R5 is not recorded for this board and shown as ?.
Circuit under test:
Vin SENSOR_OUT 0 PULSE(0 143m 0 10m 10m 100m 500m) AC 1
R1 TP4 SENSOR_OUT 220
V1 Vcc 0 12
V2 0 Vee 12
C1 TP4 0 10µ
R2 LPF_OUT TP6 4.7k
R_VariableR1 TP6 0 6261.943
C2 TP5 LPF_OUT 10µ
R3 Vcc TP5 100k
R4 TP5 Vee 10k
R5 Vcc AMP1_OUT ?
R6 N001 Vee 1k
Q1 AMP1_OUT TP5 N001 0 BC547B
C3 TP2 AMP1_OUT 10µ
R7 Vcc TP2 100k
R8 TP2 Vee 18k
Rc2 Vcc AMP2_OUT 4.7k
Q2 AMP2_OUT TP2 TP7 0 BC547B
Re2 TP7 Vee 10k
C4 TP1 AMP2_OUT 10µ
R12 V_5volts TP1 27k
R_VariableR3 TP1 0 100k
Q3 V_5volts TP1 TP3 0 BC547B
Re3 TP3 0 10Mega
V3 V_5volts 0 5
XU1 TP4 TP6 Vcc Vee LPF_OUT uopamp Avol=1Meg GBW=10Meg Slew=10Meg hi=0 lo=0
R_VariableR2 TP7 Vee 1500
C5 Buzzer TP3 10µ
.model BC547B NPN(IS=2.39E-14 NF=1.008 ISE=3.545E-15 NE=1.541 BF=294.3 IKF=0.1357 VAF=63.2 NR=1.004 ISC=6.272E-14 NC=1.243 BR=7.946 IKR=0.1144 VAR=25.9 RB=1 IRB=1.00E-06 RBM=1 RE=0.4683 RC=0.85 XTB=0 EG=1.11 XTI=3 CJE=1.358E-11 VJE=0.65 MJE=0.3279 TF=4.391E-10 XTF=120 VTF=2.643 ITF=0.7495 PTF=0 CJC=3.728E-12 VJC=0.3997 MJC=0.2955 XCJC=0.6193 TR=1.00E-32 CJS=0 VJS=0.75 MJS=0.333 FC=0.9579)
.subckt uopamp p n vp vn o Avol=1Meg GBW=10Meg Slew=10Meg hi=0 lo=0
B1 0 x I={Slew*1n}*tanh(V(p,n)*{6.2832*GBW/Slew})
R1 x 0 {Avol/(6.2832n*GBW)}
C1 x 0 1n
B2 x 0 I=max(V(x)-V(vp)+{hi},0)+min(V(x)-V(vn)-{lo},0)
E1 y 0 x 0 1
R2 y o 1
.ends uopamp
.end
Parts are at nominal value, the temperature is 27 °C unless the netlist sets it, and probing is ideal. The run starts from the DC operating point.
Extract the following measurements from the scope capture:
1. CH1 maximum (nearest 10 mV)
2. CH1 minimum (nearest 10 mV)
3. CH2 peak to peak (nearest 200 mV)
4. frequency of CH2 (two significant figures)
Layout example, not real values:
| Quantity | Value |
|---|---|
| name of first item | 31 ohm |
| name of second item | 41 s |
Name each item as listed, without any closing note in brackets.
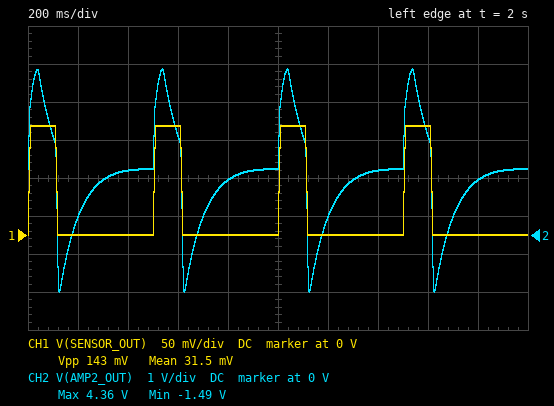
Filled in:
| Quantity | Value |
|---|---|
| CH1 maximum | 140 mV |
| CH1 minimum | 0 V |
| CH2 peak to peak | 5.8 V |
| frequency of CH2 | 2.0 Hz |
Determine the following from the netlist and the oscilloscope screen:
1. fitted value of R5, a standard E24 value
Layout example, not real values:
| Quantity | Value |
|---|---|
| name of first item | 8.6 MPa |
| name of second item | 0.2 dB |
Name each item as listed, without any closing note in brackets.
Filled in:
| Quantity | Value |
|---|---|
| fitted value of R5, a standard E24 value | 10 kΩ |
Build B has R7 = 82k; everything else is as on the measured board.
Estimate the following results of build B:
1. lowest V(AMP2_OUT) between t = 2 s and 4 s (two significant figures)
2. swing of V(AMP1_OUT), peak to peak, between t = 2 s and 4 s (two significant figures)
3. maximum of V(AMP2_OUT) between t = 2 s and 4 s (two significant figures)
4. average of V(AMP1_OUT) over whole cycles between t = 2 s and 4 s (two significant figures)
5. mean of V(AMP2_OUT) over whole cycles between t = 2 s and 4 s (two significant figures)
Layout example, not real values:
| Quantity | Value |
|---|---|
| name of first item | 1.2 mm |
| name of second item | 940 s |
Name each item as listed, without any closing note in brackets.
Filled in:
| Quantity | Value |
|---|---|
| lowest V(AMP2_OUT) between t = 2 s and 4 s | -3.7 V |
| swing of V(AMP1_OUT), peak to peak, between t = 2 s and 4 s | 2.0 V |
| maximum of V(AMP2_OUT) between t = 2 s and 4 s | 2.1 V |
| average of V(AMP1_OUT) over whole cycles between t = 2 s and 4 s | -2.9 V |
| mean of V(AMP2_OUT) over whole cycles between t = 2 s and 4 s | -680 mV |
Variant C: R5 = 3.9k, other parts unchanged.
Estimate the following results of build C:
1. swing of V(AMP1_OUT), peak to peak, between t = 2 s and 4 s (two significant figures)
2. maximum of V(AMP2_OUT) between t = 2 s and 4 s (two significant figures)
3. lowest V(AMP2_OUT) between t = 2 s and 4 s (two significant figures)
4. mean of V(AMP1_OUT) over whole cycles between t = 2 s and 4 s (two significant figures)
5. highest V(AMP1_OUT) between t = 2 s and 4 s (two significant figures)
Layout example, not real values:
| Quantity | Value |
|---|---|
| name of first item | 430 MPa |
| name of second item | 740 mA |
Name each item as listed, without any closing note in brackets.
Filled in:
| Quantity | Value |
|---|---|
| swing of V(AMP1_OUT), peak to peak, between t = 2 s and 4 s | 1.1 V |
| maximum of V(AMP2_OUT) between t = 2 s and 4 s | 3.4 V |
| lowest V(AMP2_OUT) between t = 2 s and 4 s | -140 mV |
| mean of V(AMP1_OUT) over whole cycles between t = 2 s and 4 s | 6.2 V |
| highest V(AMP1_OUT) between t = 2 s and 4 s | 6.6 V |
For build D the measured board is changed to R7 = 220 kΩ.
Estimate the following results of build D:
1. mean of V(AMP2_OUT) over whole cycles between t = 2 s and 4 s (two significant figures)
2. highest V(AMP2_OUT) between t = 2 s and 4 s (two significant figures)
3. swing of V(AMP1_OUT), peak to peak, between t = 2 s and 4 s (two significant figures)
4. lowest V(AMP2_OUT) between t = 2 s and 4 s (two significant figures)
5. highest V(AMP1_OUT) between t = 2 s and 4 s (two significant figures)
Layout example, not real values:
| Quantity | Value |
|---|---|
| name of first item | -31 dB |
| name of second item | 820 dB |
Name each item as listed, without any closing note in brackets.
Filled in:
| Quantity | Value |
|---|---|
| mean of V(AMP2_OUT) over whole cycles between t = 2 s and 4 s | 7.9 V |
| highest V(AMP2_OUT) between t = 2 s and 4 s | 11 V |
| swing of V(AMP1_OUT), peak to peak, between t = 2 s and 4 s | 2.2 V |
| lowest V(AMP2_OUT) between t = 2 s and 4 s | 4.7 V |
| highest V(AMP1_OUT) between t = 2 s and 4 s | -2.0 V |
